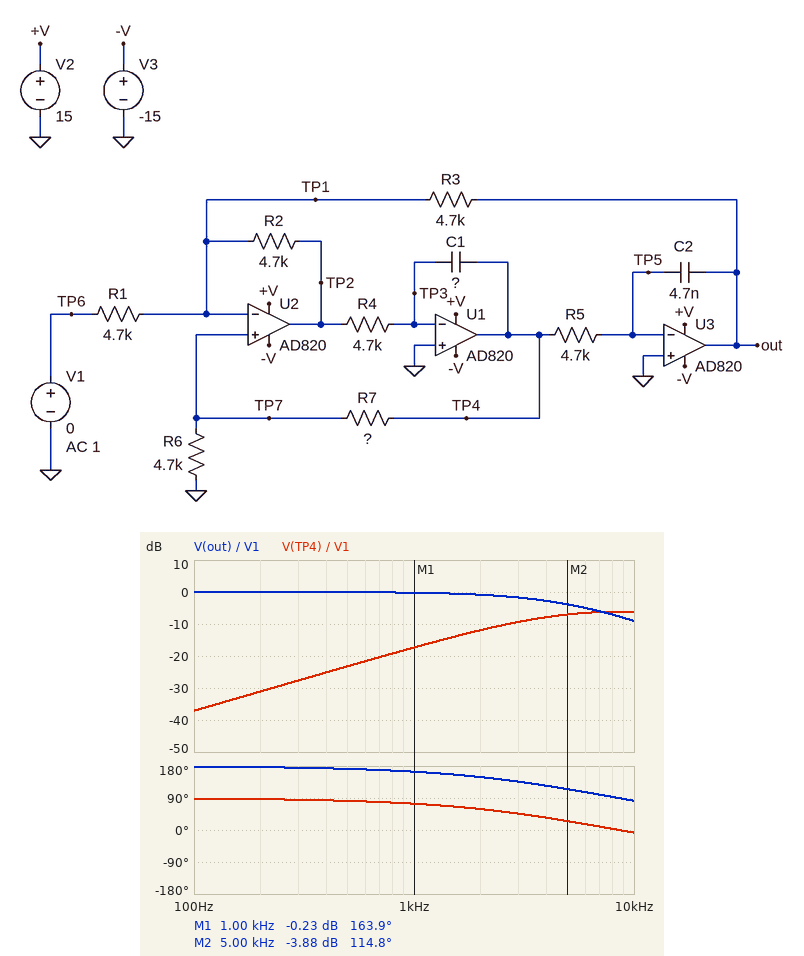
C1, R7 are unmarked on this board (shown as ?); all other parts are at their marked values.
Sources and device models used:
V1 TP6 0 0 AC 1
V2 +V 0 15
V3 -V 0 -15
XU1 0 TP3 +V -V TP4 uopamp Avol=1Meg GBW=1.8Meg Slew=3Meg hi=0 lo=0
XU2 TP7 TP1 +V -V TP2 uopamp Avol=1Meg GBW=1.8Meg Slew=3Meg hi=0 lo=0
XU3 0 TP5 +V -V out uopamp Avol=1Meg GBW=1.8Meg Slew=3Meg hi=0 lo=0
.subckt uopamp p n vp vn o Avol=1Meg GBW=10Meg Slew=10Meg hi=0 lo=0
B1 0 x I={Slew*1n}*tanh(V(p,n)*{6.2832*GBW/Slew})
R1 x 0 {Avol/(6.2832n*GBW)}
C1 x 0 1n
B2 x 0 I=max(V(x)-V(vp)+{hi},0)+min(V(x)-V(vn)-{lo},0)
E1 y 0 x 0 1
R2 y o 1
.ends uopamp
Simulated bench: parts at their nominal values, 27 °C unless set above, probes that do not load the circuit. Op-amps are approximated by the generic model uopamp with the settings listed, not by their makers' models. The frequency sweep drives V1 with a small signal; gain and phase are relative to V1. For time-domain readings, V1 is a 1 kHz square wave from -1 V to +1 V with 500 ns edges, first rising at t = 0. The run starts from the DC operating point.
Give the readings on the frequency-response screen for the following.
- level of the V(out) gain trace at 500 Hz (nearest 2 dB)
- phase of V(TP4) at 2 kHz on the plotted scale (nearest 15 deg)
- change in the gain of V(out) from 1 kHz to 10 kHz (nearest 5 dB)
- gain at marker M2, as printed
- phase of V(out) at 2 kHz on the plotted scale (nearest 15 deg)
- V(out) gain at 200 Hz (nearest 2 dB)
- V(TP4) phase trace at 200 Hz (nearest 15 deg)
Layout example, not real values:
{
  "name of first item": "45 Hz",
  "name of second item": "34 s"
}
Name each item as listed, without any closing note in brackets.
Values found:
{
  "level of the V(out) gain trace at 500 Hz": "0 dB",
  "phase of V(TP4) at 2 kHz on the plotted scale": "60 deg",
  "change in the gain of V(out) from 1 kHz to 10 kHz": "-10 dB",
  "gain at marker M2, as printed": "-3.88 dB",
  "phase of V(out) at 2 kHz on the plotted scale": "150 deg",
  "V(out) gain at 200 Hz": "0 dB",
  "V(TP4) phase trace at 200 Hz": "90 deg"
}
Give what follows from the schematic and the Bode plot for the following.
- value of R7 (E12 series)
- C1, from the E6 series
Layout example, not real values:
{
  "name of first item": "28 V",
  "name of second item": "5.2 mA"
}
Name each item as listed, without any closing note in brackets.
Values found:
{
  "value of R7": "2.2 kΩ",
  "C1, from the E6 series": "3.3 nF"
}
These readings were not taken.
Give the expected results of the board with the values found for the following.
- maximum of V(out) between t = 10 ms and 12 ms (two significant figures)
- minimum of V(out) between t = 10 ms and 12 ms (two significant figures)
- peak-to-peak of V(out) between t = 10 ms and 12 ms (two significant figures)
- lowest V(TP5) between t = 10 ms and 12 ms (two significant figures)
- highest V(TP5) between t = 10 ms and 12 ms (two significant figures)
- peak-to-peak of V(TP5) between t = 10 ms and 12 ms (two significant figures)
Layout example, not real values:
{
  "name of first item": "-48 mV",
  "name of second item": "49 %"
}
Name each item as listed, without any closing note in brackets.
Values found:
{
  "maximum of V(out) between t = 10 ms and 12 ms": "1.0 V",
  "minimum of V(out) between t = 10 ms and 12 ms": "-1.0 V",
  "peak-to-peak of V(out) between t = 10 ms and 12 ms": "2.0 V",
  "lowest V(TP5) between t = 10 ms and 12 ms": "-3.1 mV",
  "highest V(TP5) between t = 10 ms and 12 ms": "3.1 mV",
  "peak-to-peak of V(TP5) between t = 10 ms and 12 ms": "6.2 mV"
}
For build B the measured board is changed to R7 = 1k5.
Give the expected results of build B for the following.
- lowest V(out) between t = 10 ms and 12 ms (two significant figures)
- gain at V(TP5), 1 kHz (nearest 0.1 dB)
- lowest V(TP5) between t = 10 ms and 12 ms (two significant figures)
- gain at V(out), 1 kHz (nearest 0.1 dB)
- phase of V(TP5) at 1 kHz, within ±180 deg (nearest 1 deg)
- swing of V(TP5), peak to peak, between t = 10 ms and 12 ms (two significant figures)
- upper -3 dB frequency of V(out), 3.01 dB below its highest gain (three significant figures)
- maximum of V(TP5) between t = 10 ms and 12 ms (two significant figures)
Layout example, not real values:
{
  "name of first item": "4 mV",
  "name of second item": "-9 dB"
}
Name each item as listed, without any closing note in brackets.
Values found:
{
  "lowest V(out) between t = 10 ms and 12 ms": "-1.0 V",
  "gain at V(TP5), 1 kHz": "-65.4 dB",
  "lowest V(TP5) between t = 10 ms and 12 ms": "-2.9 mV",
  "gain at V(out), 1 kHz": "-0.3 dB",
  "phase of V(TP5) at 1 kHz, within ±180 deg": "72 deg",
  "swing of V(TP5), peak to peak, between t = 10 ms and 12 ms": "5.7 mV",
  "upper -3 dB frequency of V(out), 3.01 dB below its highest gain": "3.65 kHz",
  "maximum of V(TP5) between t = 10 ms and 12 ms": "2.9 mV"
}
